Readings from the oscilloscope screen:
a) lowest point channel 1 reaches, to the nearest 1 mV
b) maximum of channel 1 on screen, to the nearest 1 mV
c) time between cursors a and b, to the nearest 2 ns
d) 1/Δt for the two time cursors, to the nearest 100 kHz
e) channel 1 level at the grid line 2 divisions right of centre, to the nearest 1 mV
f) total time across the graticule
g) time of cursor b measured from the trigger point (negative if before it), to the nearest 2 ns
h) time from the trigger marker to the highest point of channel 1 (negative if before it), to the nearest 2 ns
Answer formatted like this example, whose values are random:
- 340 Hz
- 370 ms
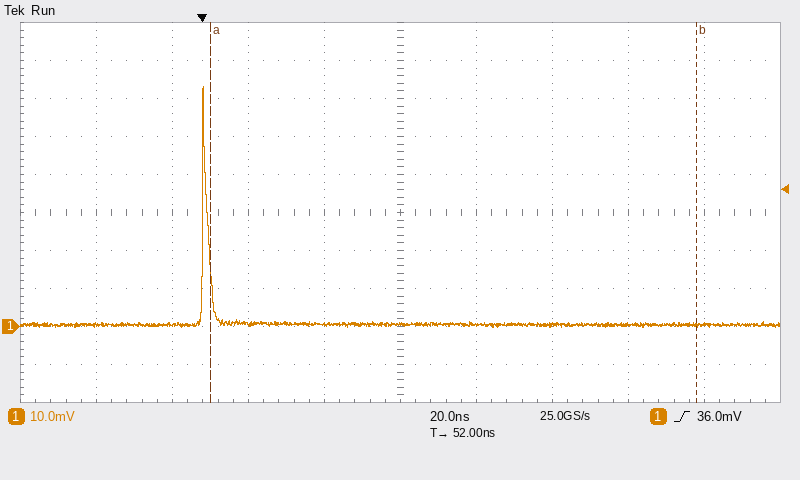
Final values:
- 0 mV
- 63 mV
- 128 ns
- 7.8 MHz
- 0 mV
- 200 ns
- +130 ns
- 0 ns
